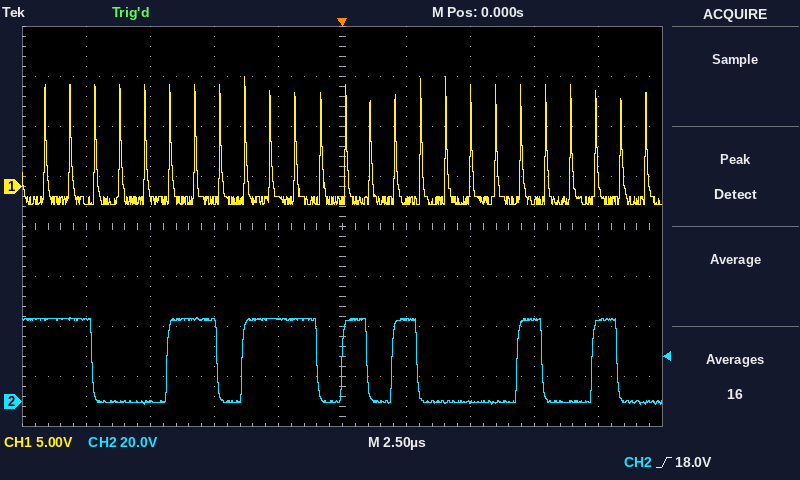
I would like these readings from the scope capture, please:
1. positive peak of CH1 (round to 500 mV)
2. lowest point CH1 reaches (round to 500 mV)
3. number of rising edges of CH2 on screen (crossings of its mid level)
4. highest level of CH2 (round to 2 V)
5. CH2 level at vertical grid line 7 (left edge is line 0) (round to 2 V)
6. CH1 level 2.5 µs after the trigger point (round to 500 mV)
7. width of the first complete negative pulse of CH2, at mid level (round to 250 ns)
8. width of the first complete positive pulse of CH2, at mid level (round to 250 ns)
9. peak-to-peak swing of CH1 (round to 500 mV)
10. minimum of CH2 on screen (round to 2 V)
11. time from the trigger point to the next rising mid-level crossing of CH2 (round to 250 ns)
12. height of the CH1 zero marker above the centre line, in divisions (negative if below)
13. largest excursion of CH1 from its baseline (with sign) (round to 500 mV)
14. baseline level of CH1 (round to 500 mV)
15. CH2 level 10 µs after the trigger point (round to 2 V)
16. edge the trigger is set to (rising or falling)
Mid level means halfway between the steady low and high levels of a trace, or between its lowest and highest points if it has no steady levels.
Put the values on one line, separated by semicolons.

11.0 V; -2.0 V; 6; 34 V; 0 V; -1.5 V; 3.00 µs; 2.00 µs; 13.0 V; -2 V; 2.00 µs; +0.8 div; +12.5 V; -1.5 V; 32 V; rising
